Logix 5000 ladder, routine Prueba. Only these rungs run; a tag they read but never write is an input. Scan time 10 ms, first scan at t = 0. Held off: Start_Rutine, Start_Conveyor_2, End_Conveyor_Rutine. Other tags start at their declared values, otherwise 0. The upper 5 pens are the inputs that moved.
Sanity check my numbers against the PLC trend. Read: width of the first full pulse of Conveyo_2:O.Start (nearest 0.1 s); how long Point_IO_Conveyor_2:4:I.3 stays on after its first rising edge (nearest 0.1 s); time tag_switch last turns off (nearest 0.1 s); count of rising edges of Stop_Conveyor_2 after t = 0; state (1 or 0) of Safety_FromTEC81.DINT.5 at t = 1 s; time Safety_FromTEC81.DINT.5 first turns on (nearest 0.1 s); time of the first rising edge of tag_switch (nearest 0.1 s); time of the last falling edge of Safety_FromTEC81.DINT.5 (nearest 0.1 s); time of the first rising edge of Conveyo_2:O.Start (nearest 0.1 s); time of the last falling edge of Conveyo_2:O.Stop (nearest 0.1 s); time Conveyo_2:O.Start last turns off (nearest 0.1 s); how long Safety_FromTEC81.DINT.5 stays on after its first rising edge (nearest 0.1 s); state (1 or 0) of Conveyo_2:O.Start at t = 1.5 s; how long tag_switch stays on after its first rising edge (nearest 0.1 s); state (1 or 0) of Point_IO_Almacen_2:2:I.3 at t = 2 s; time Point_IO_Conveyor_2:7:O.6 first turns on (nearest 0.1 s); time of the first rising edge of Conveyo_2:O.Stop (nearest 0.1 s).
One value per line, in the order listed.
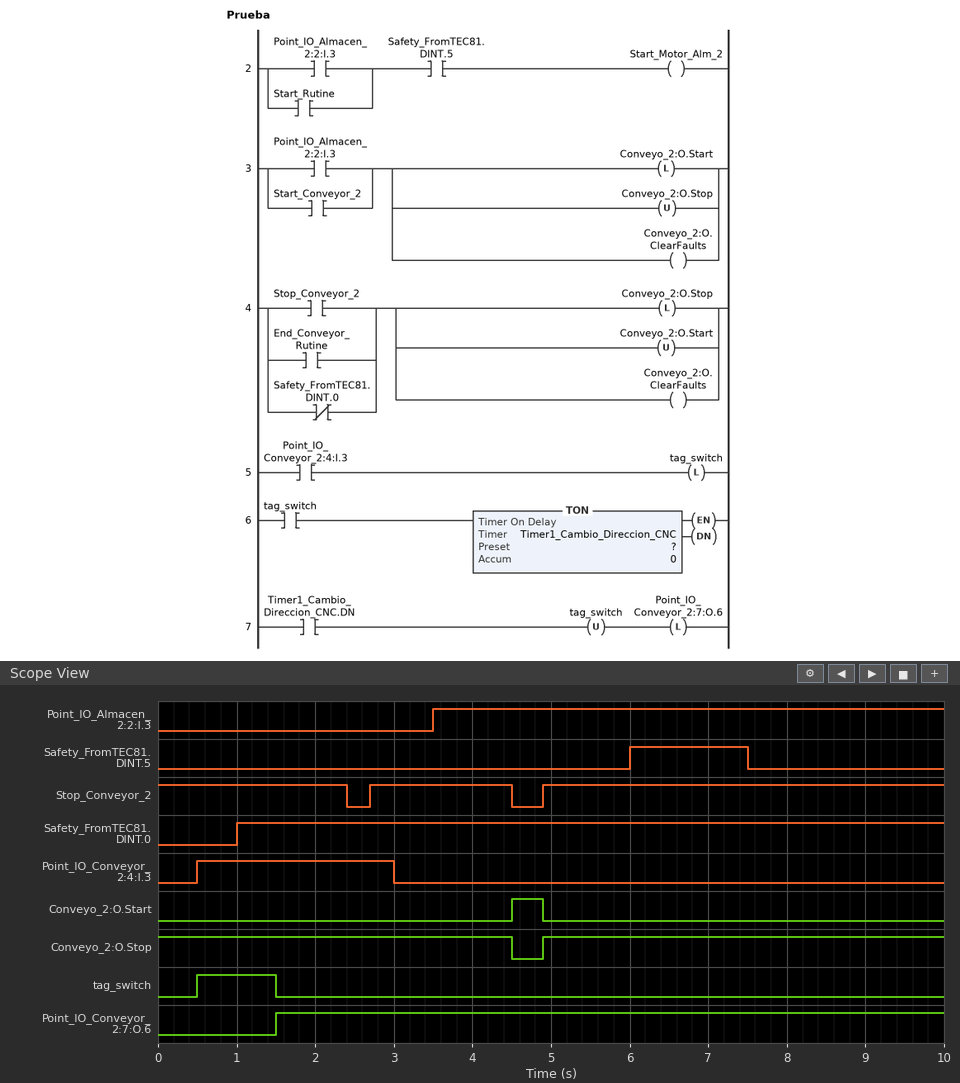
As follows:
0.4 s
2.5 s
1.5 s
2
0
6.0 s
0.5 s
7.5 s
4.5 s
4.5 s
4.9 s
1.5 s
0
1.0 s
0
1.5 s
4.9 s
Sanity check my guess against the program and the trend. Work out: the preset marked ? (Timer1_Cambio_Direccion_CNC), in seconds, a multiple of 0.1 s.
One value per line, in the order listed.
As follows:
1.0 s
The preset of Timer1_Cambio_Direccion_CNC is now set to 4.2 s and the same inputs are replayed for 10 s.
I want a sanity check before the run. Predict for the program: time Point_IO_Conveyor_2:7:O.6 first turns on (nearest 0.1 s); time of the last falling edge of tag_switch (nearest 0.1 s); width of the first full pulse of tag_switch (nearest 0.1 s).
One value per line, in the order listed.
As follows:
4.7 s
4.7 s
4.2 s
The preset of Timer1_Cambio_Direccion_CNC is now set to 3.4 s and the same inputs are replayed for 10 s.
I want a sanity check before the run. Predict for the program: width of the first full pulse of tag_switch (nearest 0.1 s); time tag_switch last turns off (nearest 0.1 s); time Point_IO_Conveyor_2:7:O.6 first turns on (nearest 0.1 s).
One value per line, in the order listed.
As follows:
3.4 s
3.9 s
3.9 s
